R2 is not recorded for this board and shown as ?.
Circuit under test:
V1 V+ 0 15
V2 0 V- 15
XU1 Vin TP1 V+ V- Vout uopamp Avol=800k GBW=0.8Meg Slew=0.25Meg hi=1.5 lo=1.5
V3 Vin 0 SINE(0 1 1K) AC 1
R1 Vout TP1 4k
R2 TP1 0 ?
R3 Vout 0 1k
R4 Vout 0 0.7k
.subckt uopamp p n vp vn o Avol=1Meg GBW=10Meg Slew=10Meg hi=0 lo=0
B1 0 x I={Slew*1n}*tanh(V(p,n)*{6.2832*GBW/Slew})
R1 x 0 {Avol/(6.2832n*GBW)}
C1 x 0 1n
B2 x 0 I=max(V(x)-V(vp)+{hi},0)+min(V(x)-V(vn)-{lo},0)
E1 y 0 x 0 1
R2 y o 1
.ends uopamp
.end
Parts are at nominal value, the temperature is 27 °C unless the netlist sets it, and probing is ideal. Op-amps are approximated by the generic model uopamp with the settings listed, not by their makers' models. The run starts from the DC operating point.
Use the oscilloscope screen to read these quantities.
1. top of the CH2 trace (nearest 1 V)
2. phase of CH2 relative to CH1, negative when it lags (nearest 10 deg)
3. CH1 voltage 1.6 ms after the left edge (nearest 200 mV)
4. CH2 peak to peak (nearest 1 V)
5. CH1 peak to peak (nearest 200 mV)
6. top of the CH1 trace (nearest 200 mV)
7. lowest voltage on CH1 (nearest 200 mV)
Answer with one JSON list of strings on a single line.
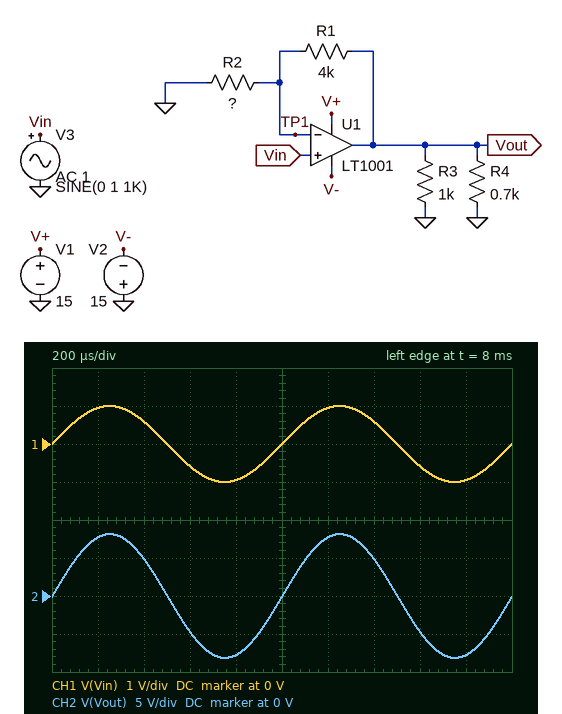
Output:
["8 V", "0 deg", "-600 mV", "16 V", "2.0 V", "1.0 V", "-1.0 V"]
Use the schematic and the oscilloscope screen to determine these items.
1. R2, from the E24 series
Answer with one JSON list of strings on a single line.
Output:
["560 Ω"]
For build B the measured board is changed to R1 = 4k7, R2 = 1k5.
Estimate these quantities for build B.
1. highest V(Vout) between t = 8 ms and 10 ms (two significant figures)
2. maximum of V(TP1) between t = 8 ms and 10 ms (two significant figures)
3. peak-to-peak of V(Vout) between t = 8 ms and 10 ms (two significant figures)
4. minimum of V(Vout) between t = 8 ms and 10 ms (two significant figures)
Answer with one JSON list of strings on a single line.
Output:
["4.1 V", "1.0 V", "8.3 V", "-4.1 V"]
